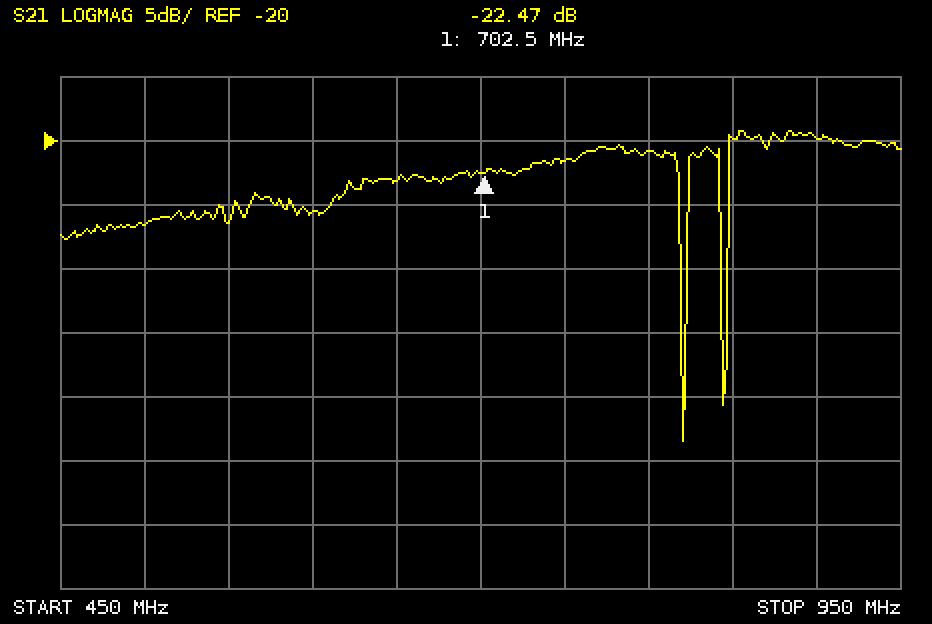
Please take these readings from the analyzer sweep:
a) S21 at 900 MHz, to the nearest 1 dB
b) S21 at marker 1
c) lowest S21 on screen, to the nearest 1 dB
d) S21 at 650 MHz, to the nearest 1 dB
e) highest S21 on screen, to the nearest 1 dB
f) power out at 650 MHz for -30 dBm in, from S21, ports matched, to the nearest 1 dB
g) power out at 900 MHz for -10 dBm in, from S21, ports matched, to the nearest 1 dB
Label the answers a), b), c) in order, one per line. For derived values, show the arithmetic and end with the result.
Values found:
a) -20 dB
b) -22.47 dB
c) -43 dB
d) -23 dB
e) -19 dB
f) -30 dBm + (-23 dB) = -53 dBm
g) -10 dBm + (-20 dB) = -30 dBm
